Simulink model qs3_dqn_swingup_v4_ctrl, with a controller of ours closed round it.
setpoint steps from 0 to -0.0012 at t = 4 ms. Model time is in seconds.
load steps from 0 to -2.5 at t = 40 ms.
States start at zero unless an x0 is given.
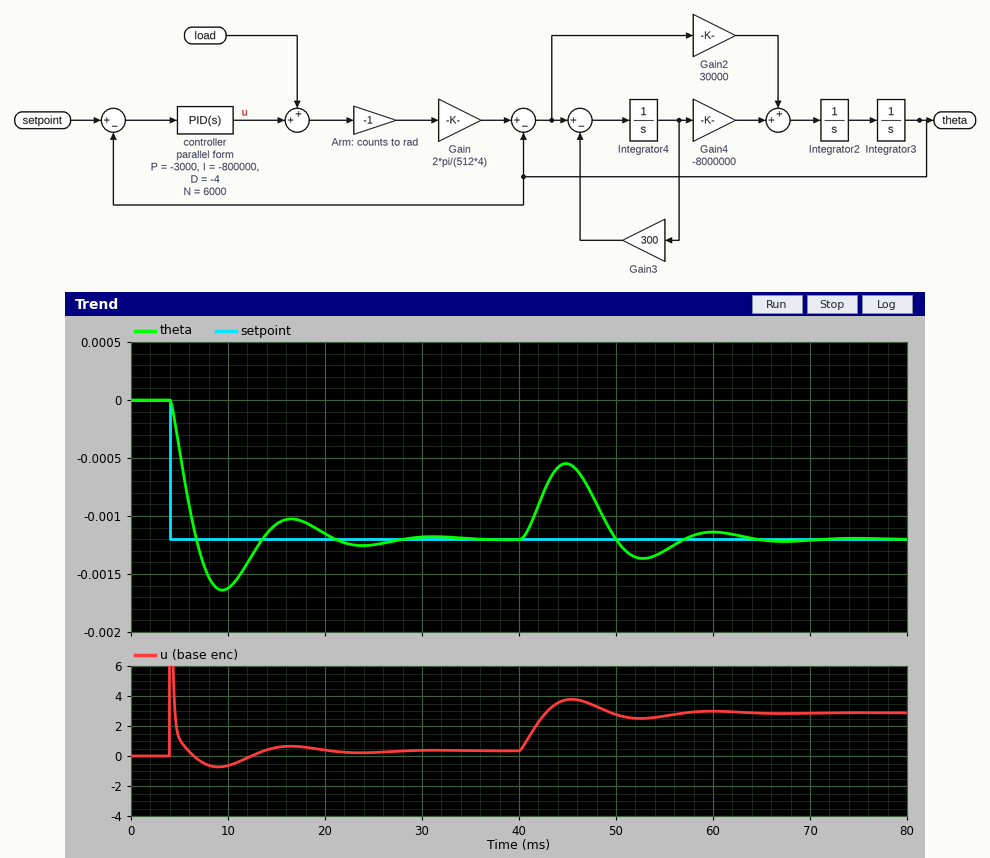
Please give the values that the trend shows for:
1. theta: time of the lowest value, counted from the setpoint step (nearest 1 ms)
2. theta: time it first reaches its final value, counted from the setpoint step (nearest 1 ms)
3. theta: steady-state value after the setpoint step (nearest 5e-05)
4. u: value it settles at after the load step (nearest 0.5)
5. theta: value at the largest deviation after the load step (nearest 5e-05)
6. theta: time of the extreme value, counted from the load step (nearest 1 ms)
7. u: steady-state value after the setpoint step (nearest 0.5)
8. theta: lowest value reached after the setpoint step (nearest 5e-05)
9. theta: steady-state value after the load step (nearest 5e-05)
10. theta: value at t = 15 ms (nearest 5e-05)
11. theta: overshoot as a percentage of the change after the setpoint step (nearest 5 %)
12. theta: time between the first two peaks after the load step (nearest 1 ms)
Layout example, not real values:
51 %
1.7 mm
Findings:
5 ms
3 ms
-0.00120
3.0
-0.00055
5 ms
0.5
-0.00165
-0.00120
-0.00105
35 %
15 ms
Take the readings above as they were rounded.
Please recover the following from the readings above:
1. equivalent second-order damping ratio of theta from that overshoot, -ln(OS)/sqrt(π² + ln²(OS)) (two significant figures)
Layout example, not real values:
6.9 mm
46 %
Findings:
0.32
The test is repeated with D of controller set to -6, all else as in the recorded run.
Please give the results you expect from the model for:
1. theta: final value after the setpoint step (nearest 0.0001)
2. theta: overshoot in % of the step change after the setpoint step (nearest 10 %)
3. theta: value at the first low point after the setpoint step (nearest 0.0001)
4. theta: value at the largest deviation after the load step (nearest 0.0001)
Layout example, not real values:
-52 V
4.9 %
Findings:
-0.0012
20 %
-0.0015
-0.0006
